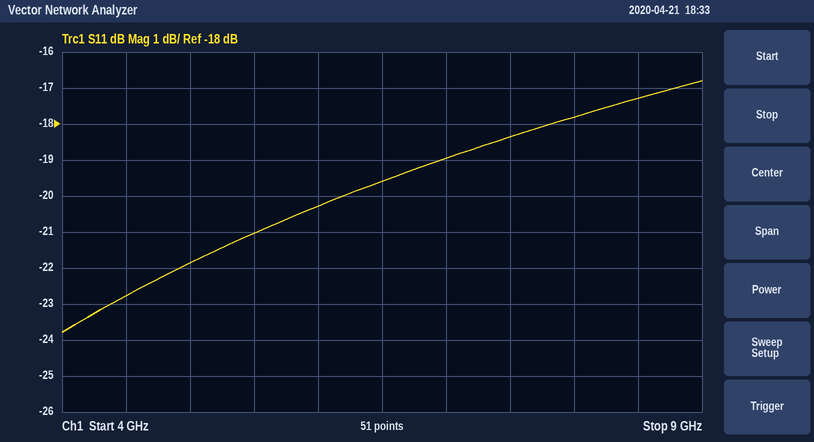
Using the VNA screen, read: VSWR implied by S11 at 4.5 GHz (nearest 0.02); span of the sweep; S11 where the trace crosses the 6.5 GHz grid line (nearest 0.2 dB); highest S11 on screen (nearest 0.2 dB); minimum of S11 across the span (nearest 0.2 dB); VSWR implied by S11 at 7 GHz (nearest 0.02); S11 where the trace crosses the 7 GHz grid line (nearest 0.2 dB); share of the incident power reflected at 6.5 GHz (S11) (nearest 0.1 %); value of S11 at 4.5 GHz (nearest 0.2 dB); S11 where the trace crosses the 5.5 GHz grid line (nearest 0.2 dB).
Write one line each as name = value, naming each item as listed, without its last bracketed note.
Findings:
VSWR implied by S11 at 4.5 GHz = 1.16
span of the sweep = 5 GHz
S11 where the trace crosses the 6.5 GHz grid line = -19.6 dB
highest S11 on screen = -16.8 dB
minimum of S11 across the span = -23.8 dB
VSWR implied by S11 at 7 GHz = 1.26
S11 where the trace crosses the 7 GHz grid line = -19.0 dB
share of the incident power reflected at 6.5 GHz (S11) = 1.1 %
value of S11 at 4.5 GHz = -22.8 dB
S11 where the trace crosses the 5.5 GHz grid line = -21.0 dB
